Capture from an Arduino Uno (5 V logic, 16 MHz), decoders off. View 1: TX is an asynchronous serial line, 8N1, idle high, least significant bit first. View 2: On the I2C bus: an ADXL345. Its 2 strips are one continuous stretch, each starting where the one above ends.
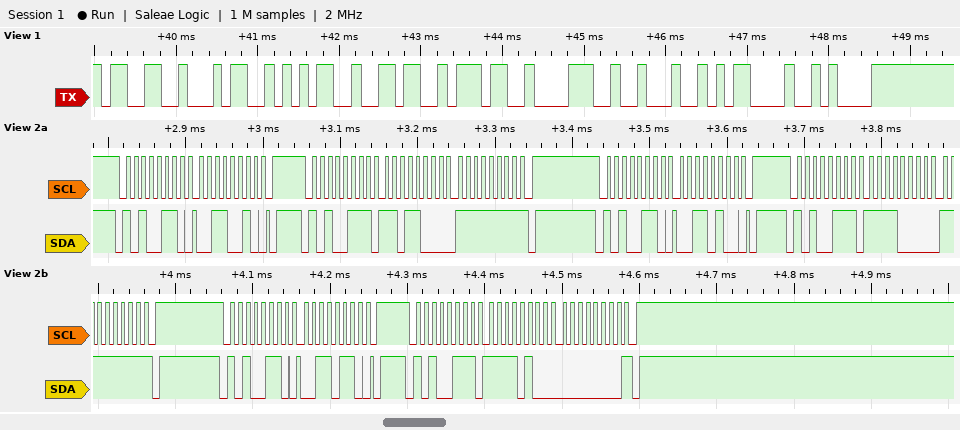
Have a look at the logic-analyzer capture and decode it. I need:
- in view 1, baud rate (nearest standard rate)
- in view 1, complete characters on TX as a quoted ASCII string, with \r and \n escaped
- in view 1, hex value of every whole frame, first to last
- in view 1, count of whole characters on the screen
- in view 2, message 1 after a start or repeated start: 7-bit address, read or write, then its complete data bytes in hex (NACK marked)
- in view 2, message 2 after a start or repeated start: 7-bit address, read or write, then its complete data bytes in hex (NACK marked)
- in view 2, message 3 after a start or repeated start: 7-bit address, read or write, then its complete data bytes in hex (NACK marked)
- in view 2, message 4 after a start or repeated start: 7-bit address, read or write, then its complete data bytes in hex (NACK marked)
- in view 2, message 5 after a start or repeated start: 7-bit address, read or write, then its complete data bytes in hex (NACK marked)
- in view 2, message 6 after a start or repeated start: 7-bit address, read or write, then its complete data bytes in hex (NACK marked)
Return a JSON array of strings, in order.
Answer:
["9600 baud", "\"345678\\\"\\r\\n\"", "33 34 35 36 37 38 22 0D 0A", "9", "0x53 write: 32", "0x53 read: D8 FF NACK", "0x53 write: 34", "0x53 read: F0 FF NACK", "0x53 write: 36", "0x53 read: F4 00 NACK"]
